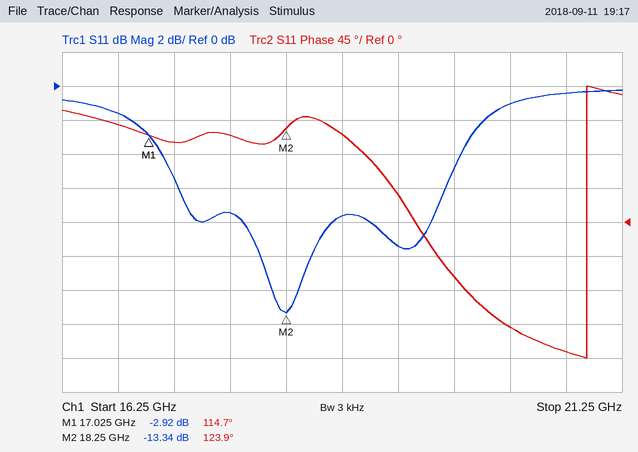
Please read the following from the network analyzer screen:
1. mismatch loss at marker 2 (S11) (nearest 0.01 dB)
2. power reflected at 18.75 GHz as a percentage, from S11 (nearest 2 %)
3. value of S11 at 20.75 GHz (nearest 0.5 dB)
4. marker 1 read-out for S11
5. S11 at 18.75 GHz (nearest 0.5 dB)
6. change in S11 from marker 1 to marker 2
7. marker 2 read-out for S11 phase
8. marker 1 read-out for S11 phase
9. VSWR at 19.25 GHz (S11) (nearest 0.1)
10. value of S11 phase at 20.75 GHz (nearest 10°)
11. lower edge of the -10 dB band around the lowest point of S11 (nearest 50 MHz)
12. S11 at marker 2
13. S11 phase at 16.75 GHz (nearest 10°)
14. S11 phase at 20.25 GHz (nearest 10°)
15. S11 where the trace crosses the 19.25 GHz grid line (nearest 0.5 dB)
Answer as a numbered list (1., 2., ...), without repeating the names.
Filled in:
1. 0.21 dB
2. 18 %
3. -0.5 dB
4. -2.92 dB
5. -7.5 dB
6. -10.42 dB
7. 123.9°
8. 114.7°
9. 2.0
10. -170°
11. 18.00 GHz
12. -13.34 dB
13. 130°
14. -140°
15. -9.5 dB
